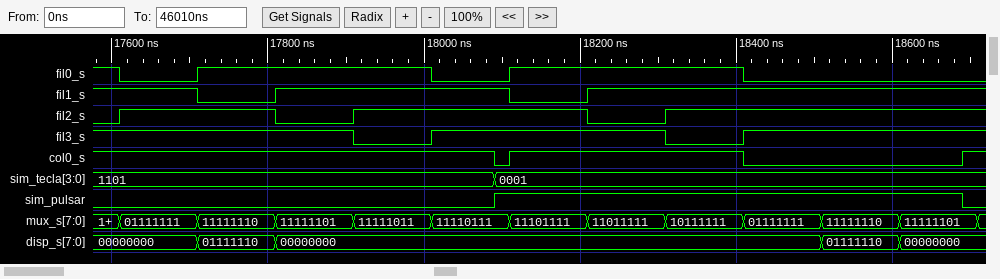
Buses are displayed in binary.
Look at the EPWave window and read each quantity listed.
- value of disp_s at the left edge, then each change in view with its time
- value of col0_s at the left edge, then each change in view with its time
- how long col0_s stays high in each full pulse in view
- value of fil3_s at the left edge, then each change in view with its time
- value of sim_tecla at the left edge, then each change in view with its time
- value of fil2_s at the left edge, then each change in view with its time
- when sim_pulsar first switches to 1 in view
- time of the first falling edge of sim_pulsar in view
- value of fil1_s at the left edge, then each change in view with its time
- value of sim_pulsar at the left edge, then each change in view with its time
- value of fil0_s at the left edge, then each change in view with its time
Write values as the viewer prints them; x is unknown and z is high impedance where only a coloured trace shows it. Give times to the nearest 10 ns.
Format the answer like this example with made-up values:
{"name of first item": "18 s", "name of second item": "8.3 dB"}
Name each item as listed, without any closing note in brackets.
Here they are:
{"value of disp_s at the left edge, then each change in view with its time": "00000000, 01111110 at 17710 ns, 00000000 at 17810 ns, 01111110 at 18510 ns, 00000000 at 18610 ns", "value of col0_s at the left edge, then each change in view with its time": "1, 0 at 18090 ns, 1 at 18110 ns, 0 at 18410 ns, 1 at 18690 ns", "how long col0_s stays high in each full pulse in view": "300 ns", "value of fil3_s at the left edge, then each change in view with its time": "1, 0 at 17910 ns, 1 at 18010 ns, 0 at 18310 ns, 1 at 18410 ns", "value of sim_tecla at the left edge, then each change in view with its time": "1101, 0001 at 18090 ns", "value of fil2_s at the left edge, then each change in view with its time": "0, 1 at 17610 ns, 0 at 17810 ns, 1 at 17910 ns, 0 at 18210 ns, 1 at 18310 ns", "when sim_pulsar first switches to 1 in view": "18090 ns", "time of the first falling edge of sim_pulsar in view": "18690 ns", "value of fil1_s at the left edge, then each change in view with its time": "1, 0 at 17710 ns, 1 at 17810 ns, 0 at 18110 ns, 1 at 18210 ns", "value of sim_pulsar at the left edge, then each change in view with its time": "0, 1 at 18090 ns, 0 at 18690 ns", "value of fil0_s at the left edge, then each change in view with its time": "1, 0 at 17610 ns, 1 at 17710 ns, 0 at 18010 ns, 1 at 18110 ns, 0 at 18410 ns"}
